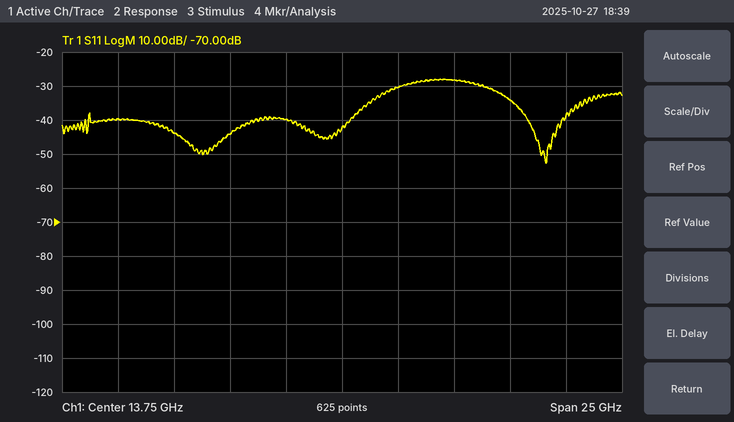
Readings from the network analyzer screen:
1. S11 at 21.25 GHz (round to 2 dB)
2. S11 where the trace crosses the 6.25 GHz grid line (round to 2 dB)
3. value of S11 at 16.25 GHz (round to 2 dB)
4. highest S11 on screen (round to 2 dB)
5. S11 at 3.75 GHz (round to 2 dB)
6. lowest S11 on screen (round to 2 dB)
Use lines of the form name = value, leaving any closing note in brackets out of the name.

S11 at 21.25 GHz = -34 dB
S11 where the trace crosses the 6.25 GHz grid line = -44 dB
value of S11 at 16.25 GHz = -30 dB
highest S11 on screen = -28 dB
S11 at 3.75 GHz = -40 dB
lowest S11 on screen = -52 dB
